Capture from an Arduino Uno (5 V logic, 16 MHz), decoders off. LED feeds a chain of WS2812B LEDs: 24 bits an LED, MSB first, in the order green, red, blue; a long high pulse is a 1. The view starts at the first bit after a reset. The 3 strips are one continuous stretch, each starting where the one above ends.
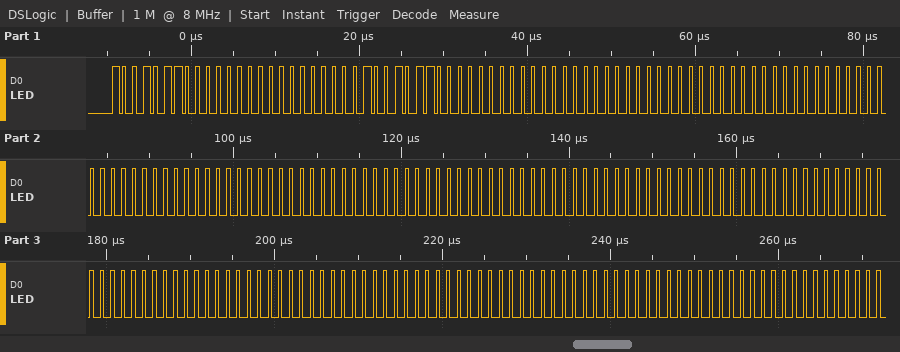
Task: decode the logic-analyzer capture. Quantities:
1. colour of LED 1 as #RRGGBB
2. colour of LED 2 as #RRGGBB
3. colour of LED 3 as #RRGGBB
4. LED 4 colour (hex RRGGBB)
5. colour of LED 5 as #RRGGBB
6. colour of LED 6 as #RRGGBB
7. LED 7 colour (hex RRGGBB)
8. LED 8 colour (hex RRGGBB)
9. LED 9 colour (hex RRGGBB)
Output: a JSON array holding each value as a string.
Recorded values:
["#009600", "#009600", "#000000", "#000000", "#000000", "#000000", "#000000", "#000000", "#000000"]
